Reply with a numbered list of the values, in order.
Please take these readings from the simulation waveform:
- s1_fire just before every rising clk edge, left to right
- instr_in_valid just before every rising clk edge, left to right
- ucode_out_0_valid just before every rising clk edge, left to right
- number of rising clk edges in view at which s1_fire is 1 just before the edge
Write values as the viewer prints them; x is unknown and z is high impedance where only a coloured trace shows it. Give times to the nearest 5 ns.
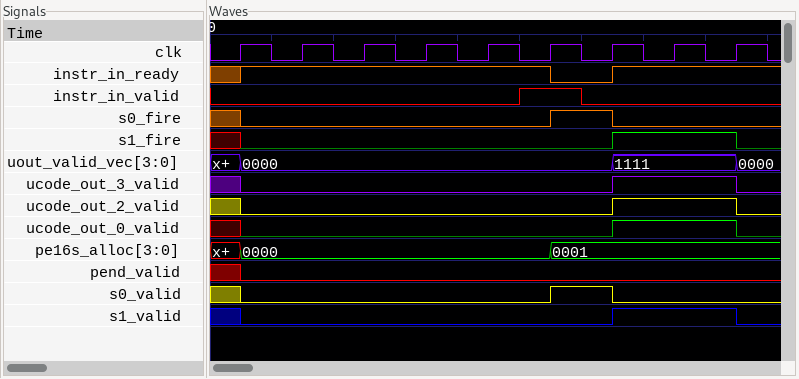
1. x 0 0 0 0 0 0 1 1
2. 0 0 0 0 0 1 0 0 0
3. x 0 0 0 0 0 0 1 1
4. 2
